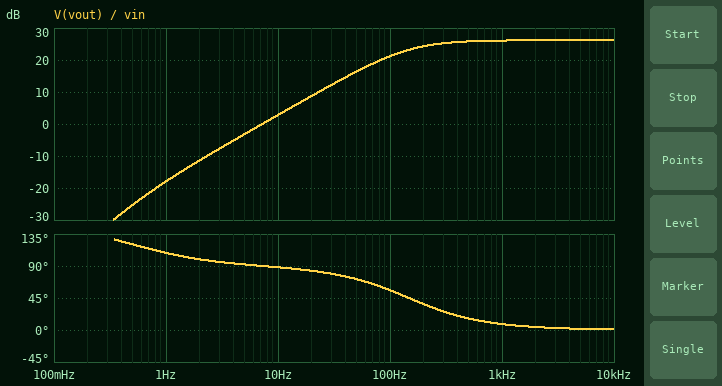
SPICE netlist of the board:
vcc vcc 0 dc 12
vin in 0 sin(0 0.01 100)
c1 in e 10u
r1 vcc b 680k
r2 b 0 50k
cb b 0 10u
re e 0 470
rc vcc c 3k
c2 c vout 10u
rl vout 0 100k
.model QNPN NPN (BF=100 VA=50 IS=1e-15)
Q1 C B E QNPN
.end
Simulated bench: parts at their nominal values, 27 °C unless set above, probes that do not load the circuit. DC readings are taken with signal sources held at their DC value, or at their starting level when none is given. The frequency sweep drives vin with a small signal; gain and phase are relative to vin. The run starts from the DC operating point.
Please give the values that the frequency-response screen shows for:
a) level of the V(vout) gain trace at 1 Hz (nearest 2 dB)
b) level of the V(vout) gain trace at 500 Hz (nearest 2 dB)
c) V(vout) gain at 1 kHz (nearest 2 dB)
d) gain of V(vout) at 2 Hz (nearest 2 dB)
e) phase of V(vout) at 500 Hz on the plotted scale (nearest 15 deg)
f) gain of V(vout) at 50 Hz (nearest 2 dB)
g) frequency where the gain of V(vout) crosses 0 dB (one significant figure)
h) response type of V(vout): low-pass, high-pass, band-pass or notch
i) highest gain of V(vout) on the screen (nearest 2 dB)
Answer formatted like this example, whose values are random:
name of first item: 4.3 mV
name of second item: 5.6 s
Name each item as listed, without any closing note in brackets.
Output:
level of the V(vout) gain trace at 1 Hz: -18 dB
level of the V(vout) gain trace at 500 Hz: 26 dB
V(vout) gain at 1 kHz: 26 dB
gain of V(vout) at 2 Hz: -12 dB
phase of V(vout) at 500 Hz on the plotted scale: 15 deg
gain of V(vout) at 50 Hz: 16 dB
frequency where the gain of V(vout) crosses 0 dB: 7 Hz
response type of V(vout): low-pass, high-pass, band-pass or notch: high-pass
highest gain of V(vout) on the screen: 26 dB
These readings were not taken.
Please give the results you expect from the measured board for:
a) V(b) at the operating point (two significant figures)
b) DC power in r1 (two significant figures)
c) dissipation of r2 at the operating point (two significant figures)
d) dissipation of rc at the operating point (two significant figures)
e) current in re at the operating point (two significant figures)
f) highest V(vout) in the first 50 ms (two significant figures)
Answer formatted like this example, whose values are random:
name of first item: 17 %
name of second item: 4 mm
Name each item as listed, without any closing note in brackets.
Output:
V(b) at the operating point: 750 mV
DC power in r1: 190 µW
dissipation of r2 at the operating point: 11 µW
dissipation of rc at the operating point: 100 µW
current in re at the operating point: 180 µA
highest V(vout) in the first 50 ms: 110 mV
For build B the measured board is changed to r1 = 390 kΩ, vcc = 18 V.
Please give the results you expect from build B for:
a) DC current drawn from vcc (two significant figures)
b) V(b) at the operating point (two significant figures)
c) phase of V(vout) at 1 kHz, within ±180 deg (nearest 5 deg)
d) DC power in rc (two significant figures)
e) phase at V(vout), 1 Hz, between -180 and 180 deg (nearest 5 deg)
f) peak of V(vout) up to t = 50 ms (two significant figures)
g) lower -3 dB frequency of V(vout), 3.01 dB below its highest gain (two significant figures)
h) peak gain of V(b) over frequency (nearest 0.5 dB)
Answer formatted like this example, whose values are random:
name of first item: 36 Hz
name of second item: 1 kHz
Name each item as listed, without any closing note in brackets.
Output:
DC current drawn from vcc: 1.6 mA
V(b) at the operating point: 1.5 V
phase of V(vout) at 1 kHz, within ±180 deg: 45 deg
DC power in rc: 7.6 mW
phase at V(vout), 1 Hz, between -180 and 180 deg: 110 deg
peak of V(vout) up to t = 50 ms: 170 mV
lower -3 dB frequency of V(vout), 3.01 dB below its highest gain: 960 Hz
peak gain of V(b) over frequency: -41.5 dB
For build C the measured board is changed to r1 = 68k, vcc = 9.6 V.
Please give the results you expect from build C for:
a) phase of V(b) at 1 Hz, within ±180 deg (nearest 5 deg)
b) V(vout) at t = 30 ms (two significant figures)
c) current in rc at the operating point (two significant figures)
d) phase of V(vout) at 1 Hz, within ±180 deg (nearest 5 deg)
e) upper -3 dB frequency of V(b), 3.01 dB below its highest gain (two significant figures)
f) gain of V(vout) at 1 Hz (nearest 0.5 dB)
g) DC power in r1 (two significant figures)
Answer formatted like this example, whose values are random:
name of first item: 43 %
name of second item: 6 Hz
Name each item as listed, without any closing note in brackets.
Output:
phase of V(b) at 1 Hz, within ±180 deg: 85 deg
V(vout) at t = 30 ms: 25 mV
current in rc at the operating point: 2.7 mA
phase of V(vout) at 1 Hz, within ±180 deg: 100 deg
upper -3 dB frequency of V(b), 3.01 dB below its highest gain: 1.8 kHz
gain of V(vout) at 1 Hz: -32.0 dB
DC power in r1: 840 µW
